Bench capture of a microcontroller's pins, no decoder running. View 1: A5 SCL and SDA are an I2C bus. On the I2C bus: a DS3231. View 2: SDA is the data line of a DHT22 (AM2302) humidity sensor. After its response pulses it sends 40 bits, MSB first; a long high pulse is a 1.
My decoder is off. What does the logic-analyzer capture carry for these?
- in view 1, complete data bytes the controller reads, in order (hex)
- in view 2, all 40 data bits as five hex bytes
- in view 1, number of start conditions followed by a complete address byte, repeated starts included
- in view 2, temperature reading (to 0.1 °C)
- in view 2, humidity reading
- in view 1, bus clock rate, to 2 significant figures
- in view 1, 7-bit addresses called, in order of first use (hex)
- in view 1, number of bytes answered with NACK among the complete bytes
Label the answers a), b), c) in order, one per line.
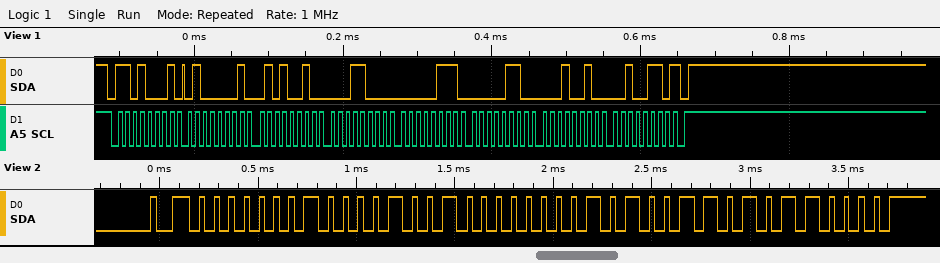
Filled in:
a) 41 52 18 07 06 12 26
b) 01 09 00 A6 B0
c) 1
d) 16.6 °C
e) 26.5 %
f) 100 kHz
g) 0x68
h) 1
